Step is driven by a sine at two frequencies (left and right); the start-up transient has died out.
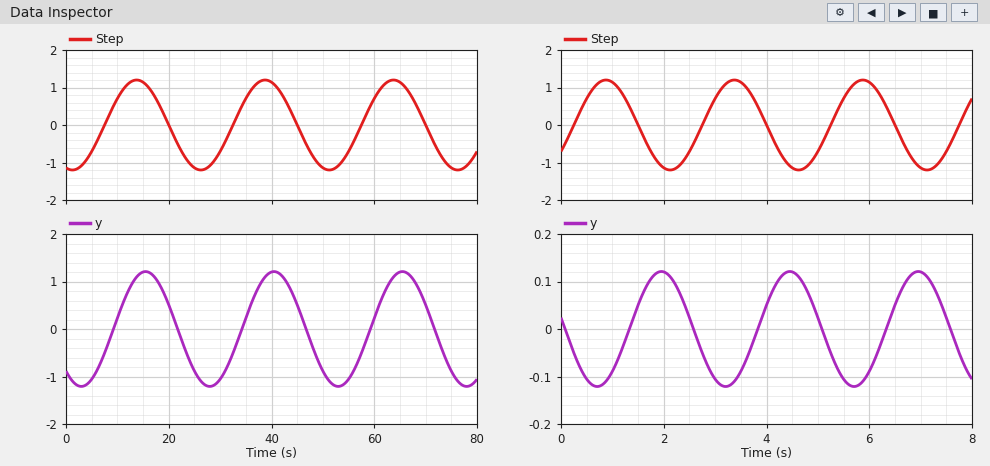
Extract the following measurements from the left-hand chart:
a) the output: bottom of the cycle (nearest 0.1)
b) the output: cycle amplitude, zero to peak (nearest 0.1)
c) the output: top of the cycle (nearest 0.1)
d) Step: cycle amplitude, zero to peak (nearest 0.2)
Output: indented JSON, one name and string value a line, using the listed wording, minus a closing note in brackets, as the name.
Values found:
{
  "the output: bottom of the cycle": "-1.2",
  "the output: cycle amplitude, zero to peak": "1.2",
  "the output: top of the cycle": "1.2",
  "Step: cycle amplitude, zero to peak": "1.2"
}
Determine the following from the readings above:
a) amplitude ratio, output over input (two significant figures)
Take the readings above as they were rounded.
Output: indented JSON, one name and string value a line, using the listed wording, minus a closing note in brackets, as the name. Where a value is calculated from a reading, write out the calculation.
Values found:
{
  "amplitude ratio, output over input": "1.2 / 1.2 = 1.0"
}
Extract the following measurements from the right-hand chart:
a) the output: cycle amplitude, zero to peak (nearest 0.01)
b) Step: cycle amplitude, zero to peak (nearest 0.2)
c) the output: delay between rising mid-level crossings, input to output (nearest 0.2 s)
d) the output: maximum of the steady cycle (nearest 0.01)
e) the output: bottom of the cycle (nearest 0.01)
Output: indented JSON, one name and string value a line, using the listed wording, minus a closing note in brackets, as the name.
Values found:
{
  "the output: cycle amplitude, zero to peak": "0.12",
  "Step: cycle amplitude, zero to peak": "1.2",
  "the output: delay between rising mid-level crossings, input to output": "1.0 s",
  "the output: maximum of the steady cycle": "0.12",
  "the output: bottom of the cycle": "-0.12"
}
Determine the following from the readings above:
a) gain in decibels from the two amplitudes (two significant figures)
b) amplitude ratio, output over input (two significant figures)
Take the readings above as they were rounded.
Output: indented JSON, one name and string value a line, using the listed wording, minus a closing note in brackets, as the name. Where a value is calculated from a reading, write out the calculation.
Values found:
{
  "gain in decibels from the two amplitudes": "20 log10(0.12 / 1.2) = -20 dB",
  "amplitude ratio, output over input": "0.12 / 1.2 = 0.10"
}
